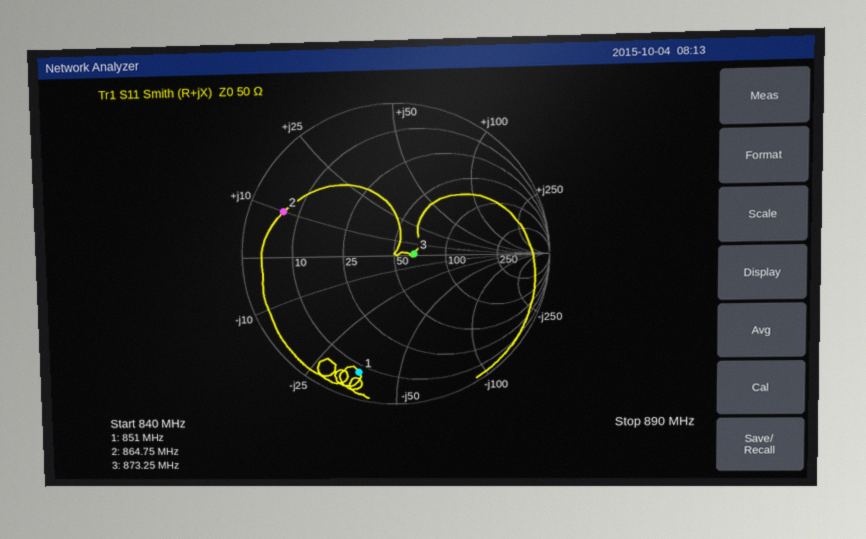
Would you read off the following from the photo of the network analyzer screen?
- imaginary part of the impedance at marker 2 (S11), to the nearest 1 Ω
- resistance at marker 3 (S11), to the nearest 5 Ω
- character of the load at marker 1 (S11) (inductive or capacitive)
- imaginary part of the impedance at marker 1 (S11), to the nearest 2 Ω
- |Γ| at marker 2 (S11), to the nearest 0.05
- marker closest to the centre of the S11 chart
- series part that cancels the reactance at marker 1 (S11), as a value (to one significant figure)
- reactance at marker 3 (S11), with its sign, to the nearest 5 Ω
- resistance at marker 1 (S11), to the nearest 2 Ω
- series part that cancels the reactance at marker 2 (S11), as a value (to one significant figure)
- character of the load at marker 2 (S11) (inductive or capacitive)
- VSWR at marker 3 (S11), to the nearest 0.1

+10 Ω
65 Ω
capacitive
-36 Ω
0.80
marker 3
7 nH
0 Ω
8 Ω
20 pF
inductive
1.3
